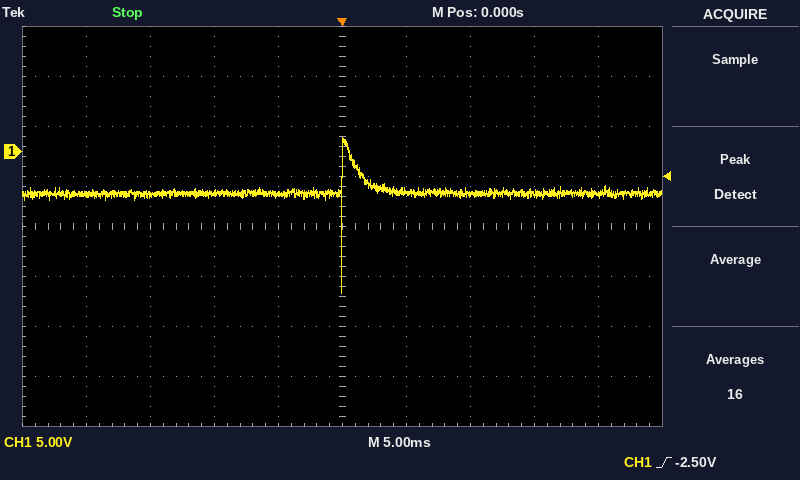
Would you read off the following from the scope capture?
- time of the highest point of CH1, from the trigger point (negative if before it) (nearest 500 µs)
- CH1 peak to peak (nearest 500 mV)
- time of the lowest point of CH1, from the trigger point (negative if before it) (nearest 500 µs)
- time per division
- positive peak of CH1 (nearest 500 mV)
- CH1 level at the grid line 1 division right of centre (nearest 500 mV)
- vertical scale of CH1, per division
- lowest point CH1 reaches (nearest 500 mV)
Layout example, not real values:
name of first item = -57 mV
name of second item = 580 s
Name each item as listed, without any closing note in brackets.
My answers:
time of the highest point of CH1, from the trigger point (negative if before it) = 0.0 ms
CH1 peak to peak = 15.5 V
time of the lowest point of CH1, from the trigger point (negative if before it) = 0.0 ms
time per division = 5 ms
positive peak of CH1 = 1.5 V
CH1 level at the grid line 1 division right of centre = -4.0 V
vertical scale of CH1, per division = 5 V
lowest point CH1 reaches = -14.0 V
